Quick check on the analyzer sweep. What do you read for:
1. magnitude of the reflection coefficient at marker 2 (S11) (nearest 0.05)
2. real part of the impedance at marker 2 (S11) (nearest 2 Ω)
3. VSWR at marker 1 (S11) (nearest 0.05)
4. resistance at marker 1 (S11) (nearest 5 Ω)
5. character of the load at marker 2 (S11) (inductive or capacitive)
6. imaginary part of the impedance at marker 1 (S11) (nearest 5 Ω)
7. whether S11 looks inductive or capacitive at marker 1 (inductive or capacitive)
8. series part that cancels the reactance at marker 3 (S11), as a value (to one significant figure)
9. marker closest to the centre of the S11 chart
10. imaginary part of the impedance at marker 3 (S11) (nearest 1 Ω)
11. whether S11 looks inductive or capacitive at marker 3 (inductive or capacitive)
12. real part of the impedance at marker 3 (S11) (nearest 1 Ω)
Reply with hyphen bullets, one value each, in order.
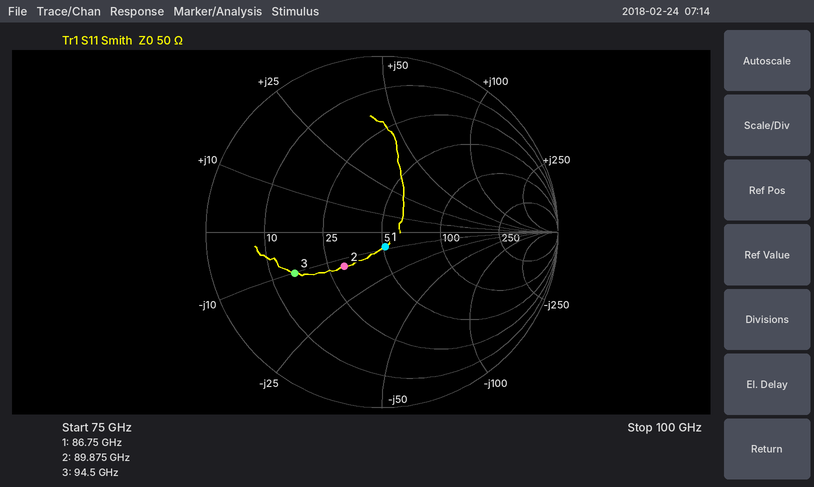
- 0.30
- 30 Ω
- 1.20
- 50 Ω
- capacitive
- -10 Ω
- capacitive
- 20 pH
- marker 1
- -10 Ω
- capacitive
- 15 Ω
